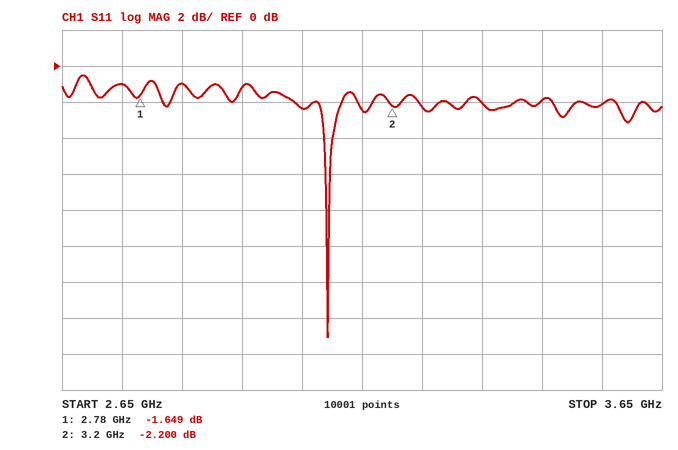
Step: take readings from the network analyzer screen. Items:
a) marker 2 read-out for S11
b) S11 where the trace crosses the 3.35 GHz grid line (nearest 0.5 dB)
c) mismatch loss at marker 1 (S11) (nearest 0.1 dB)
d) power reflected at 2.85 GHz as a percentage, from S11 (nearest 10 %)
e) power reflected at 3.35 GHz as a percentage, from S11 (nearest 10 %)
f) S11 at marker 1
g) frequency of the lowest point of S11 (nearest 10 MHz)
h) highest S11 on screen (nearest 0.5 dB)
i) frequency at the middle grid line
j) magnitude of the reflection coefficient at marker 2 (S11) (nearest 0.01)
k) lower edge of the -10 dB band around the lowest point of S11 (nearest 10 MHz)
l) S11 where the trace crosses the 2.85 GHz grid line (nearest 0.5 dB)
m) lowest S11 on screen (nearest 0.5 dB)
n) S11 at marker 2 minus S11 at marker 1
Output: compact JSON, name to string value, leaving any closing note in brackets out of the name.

{"marker 2 read-out for S11": "-2.200 dB", "S11 where the trace crosses the 3.35 GHz grid line": "-2.0 dB", "mismatch loss at marker 1 (S11)": "5.0 dB", "power reflected at 2.85 GHz as a percentage, from S11": "80 %", "power reflected at 3.35 GHz as a percentage, from S11": "60 %", "S11 at marker 1": "-1.649 dB", "frequency of the lowest point of S11": "3.09 GHz", "highest S11 on screen": "-0.5 dB", "frequency at the middle grid line": "3.15 GHz", "magnitude of the reflection coefficient at marker 2 (S11)": "0.78", "lower edge of the -10 dB band around the lowest point of S11": "3.09 GHz", "S11 where the trace crosses the 2.85 GHz grid line": "-1.0 dB", "lowest S11 on screen": "-15.0 dB", "S11 at marker 2 minus S11 at marker 1": "-0.551 dB"}
